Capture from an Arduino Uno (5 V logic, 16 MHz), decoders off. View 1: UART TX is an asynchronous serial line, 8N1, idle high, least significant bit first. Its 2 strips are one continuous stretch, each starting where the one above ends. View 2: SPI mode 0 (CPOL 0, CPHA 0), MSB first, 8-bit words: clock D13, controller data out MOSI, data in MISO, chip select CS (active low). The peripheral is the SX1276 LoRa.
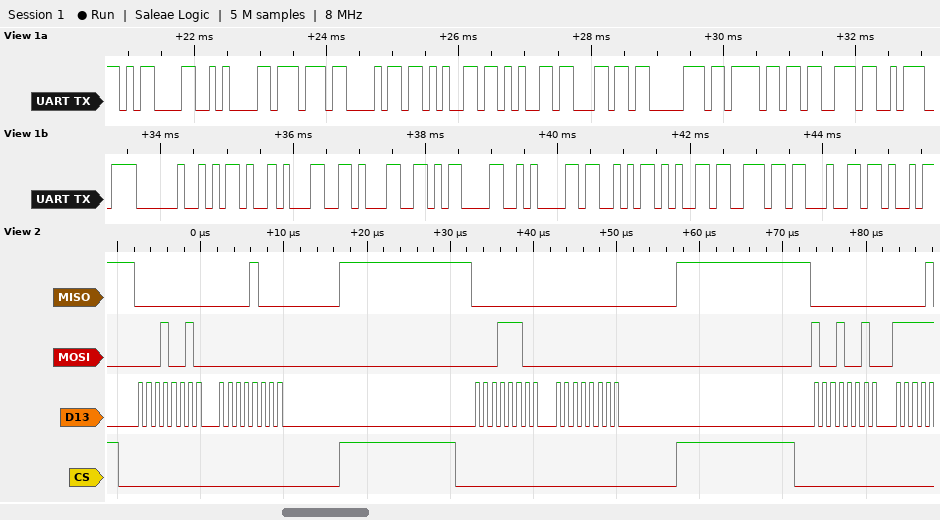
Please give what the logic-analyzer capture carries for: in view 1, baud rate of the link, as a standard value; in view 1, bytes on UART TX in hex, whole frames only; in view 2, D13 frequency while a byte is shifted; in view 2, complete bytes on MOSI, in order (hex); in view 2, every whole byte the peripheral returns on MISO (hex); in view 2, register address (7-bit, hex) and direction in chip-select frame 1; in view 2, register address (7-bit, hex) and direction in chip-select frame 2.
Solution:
9600 baud
0x0D 0x0A 0x77 0x68 0x65 0x65 0x6C 0x70 0x6F 0x73 0x3A 0x20 0x2D 0x31 0x31 0x0D 0x0A 0x53 0x65 0x6E 0x64
1 MHz
12 00 1C 00 92
00 08 00 00 00
0x12 read
0x1C read
